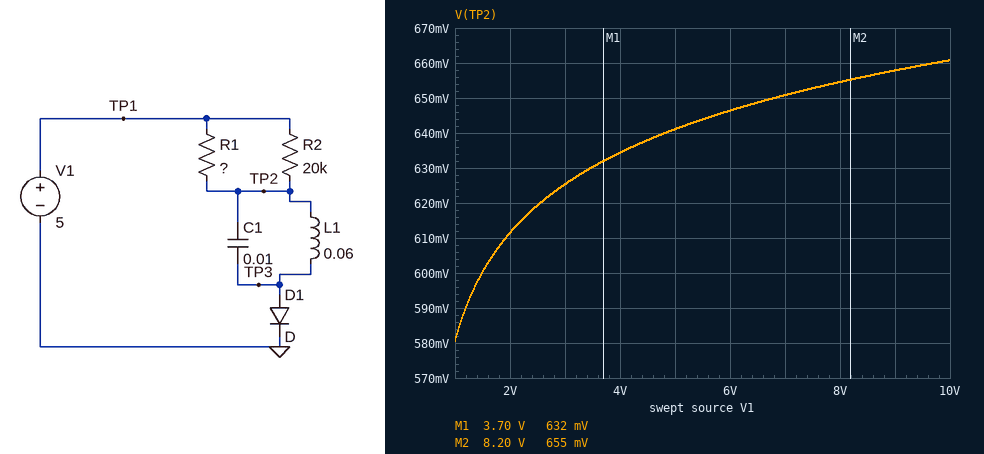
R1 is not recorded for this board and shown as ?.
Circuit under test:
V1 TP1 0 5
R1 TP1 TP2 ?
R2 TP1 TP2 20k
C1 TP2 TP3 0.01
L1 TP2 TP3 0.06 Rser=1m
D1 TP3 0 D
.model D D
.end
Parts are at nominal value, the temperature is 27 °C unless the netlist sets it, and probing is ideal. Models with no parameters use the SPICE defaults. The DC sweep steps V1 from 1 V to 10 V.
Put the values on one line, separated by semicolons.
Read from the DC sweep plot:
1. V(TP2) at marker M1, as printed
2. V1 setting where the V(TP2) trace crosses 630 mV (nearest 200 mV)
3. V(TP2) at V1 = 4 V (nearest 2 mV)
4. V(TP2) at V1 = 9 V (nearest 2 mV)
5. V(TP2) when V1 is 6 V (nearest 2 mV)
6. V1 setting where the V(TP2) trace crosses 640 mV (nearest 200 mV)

632 mV; 3.4 V; 634 mV; 658 mV; 646 mV; 4.8 V
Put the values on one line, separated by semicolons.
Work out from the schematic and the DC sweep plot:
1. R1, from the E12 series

12 kΩ
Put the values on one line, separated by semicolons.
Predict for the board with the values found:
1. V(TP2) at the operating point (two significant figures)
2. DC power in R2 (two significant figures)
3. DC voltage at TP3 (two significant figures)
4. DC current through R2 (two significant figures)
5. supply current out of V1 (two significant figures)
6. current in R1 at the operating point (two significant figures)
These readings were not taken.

640 mV; 950 µW; 640 mV; 220 µA; 580 µA; 360 µA
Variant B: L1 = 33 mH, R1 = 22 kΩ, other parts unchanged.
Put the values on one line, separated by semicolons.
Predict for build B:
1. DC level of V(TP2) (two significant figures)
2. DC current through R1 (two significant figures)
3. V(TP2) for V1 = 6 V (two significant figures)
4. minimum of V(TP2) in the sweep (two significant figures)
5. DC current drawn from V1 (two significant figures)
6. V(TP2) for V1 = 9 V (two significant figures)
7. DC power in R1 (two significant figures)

630 mV; 200 µA; 640 mV; 570 mV; 420 µA; 650 mV; 870 µW
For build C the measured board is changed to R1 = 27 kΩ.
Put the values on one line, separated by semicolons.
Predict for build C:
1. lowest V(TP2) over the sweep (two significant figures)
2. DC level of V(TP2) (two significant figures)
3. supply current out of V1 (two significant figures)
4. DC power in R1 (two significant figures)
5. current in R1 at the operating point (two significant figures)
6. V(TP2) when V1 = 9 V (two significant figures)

570 mV; 630 mV; 380 µA; 710 µW; 160 µA; 650 mV
